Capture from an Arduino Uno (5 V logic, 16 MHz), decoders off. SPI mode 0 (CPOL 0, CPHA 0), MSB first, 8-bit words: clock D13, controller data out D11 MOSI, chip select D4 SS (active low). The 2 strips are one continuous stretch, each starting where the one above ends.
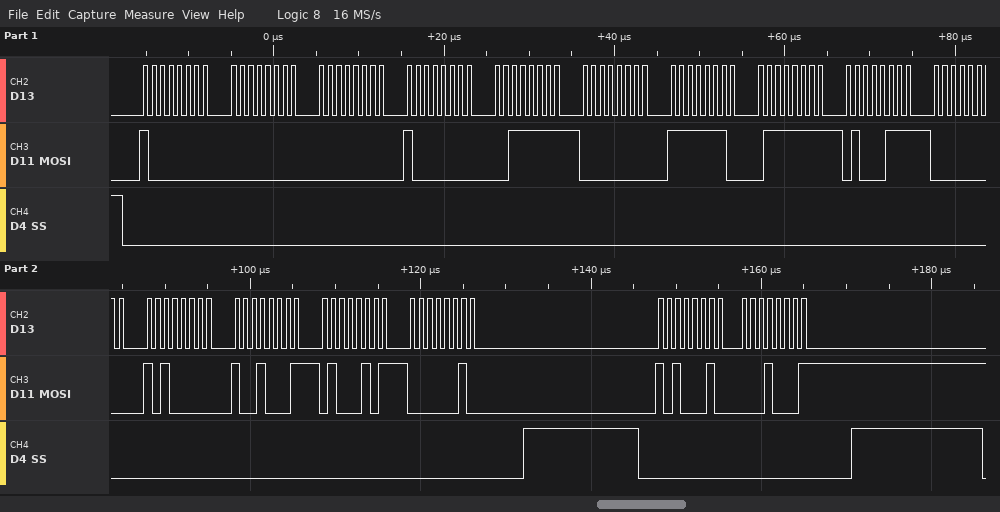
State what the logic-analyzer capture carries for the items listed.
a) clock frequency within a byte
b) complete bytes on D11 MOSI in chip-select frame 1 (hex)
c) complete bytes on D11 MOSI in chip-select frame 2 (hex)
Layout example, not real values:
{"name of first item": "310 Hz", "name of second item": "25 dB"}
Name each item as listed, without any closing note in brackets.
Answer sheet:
{"clock frequency within a byte": "1 MHz", "complete bytes on D11 MOSI in chip-select frame 1": "80 00 00 80 3F 00 FE 7F 47 00 A0 91 45 02", "complete bytes on D11 MOSI in chip-select frame 2": "A2 11"}
